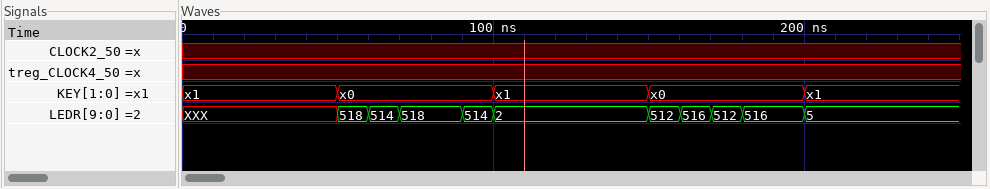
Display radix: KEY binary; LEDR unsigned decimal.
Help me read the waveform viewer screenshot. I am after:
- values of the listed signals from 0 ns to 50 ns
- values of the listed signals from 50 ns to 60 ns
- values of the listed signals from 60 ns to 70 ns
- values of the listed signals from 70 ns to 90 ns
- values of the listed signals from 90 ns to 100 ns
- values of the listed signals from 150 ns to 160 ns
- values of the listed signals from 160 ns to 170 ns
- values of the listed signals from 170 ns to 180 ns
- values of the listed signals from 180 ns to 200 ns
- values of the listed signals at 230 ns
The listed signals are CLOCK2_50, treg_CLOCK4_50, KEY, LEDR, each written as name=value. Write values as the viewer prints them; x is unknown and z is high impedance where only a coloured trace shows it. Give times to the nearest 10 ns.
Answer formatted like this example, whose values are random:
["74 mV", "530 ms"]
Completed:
["CLOCK2_50=x, treg_CLOCK4_50=x, KEY=x1, LEDR=XXX", "CLOCK2_50=x, treg_CLOCK4_50=x, KEY=x0, LEDR=518", "CLOCK2_50=x, treg_CLOCK4_50=x, KEY=x0, LEDR=514", "CLOCK2_50=x, treg_CLOCK4_50=x, KEY=x0, LEDR=518", "CLOCK2_50=x, treg_CLOCK4_50=x, KEY=x0, LEDR=514", "CLOCK2_50=x, treg_CLOCK4_50=x, KEY=x0, LEDR=512", "CLOCK2_50=x, treg_CLOCK4_50=x, KEY=x0, LEDR=516", "CLOCK2_50=x, treg_CLOCK4_50=x, KEY=x0, LEDR=512", "CLOCK2_50=x, treg_CLOCK4_50=x, KEY=x0, LEDR=516", "CLOCK2_50=x, treg_CLOCK4_50=x, KEY=x1, LEDR=5"]
